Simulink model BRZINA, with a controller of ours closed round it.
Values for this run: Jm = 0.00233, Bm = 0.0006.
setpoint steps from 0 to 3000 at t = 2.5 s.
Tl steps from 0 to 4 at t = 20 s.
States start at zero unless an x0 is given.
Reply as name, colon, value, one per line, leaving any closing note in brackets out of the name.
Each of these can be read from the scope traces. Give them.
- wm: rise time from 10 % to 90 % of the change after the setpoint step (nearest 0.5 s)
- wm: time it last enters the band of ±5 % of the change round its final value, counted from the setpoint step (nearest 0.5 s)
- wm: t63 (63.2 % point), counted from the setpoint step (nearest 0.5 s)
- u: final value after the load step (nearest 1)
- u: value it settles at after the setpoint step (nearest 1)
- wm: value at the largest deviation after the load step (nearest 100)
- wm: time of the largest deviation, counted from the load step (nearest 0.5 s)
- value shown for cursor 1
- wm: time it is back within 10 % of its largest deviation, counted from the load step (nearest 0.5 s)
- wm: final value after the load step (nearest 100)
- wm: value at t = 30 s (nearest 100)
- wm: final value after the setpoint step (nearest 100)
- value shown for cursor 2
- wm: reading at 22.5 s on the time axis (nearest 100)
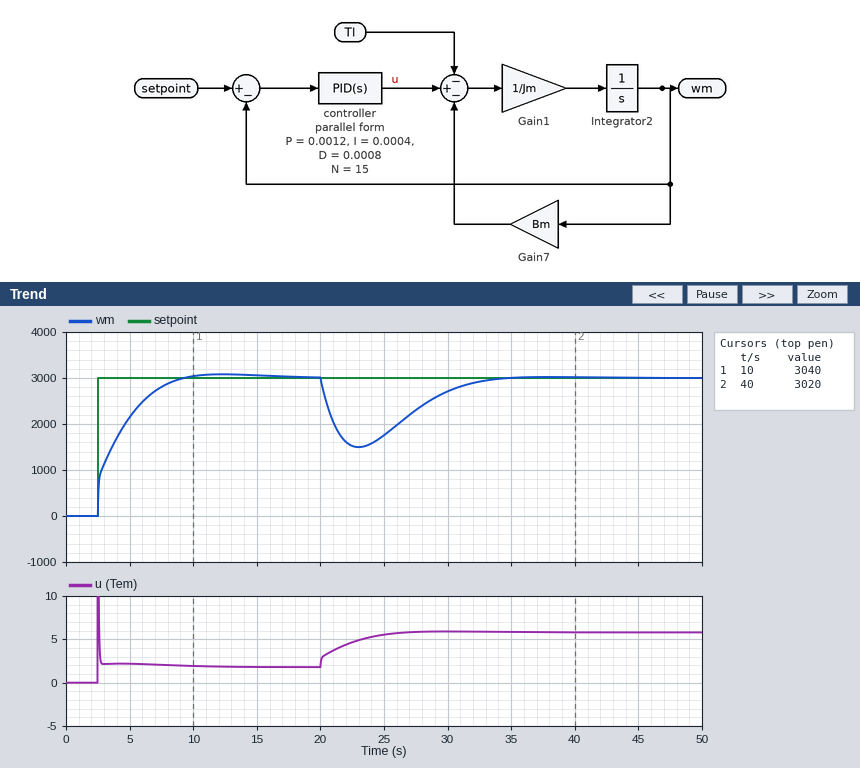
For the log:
wm: rise time from 10 % to 90 % of the change after the setpoint step: 4.5 s
wm: time it last enters the band of ±5 % of the change round its final value, counted from the setpoint step: 5.5 s
wm: t63 (63.2 % point), counted from the setpoint step: 2.0 s
u: final value after the load step: 6
u: value it settles at after the setpoint step: 2
wm: value at the largest deviation after the load step: 1500
wm: time of the largest deviation, counted from the load step: 3.0 s
value shown for cursor 1: 3040
wm: time it is back within 10 % of its largest deviation, counted from the load step: 11.5 s
wm: final value after the load step: 3000
wm: value at t = 30 s: 2700
wm: final value after the setpoint step: 3000
value shown for cursor 2: 3020
wm: reading at 22.5 s on the time axis: 1500
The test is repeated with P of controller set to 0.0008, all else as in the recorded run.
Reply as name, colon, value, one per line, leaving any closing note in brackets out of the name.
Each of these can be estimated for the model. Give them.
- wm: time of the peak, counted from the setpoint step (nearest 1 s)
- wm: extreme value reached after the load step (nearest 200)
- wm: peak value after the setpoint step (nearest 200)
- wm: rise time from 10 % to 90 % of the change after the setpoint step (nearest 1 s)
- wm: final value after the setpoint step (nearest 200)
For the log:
wm: time of the peak, counted from the setpoint step: 9 s
wm: extreme value reached after the load step: 1200
wm: peak value after the setpoint step: 3200
wm: rise time from 10 % to 90 % of the change after the setpoint step: 5 s
wm: final value after the setpoint step: 3000
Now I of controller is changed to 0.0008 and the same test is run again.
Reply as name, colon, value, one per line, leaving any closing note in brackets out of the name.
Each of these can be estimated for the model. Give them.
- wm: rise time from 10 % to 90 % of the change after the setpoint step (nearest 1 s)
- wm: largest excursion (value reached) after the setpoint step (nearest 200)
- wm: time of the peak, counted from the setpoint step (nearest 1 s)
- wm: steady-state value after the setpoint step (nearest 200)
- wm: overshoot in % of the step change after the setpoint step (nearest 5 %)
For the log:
wm: rise time from 10 % to 90 % of the change after the setpoint step: 3 s
wm: largest excursion (value reached) after the setpoint step: 3400
wm: time of the peak, counted from the setpoint step: 6 s
wm: steady-state value after the setpoint step: 3000
wm: overshoot in % of the step change after the setpoint step: 10 %
